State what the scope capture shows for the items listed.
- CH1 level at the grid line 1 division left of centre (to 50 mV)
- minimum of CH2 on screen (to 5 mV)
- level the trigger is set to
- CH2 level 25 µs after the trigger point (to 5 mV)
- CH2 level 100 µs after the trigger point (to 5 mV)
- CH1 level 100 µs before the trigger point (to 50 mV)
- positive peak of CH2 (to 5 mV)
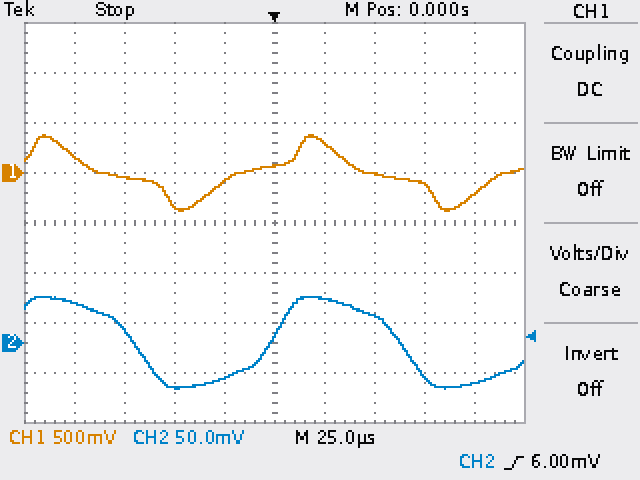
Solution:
-100 mV
-45 mV
6.00 mV
45 mV
-40 mV
150 mV
45 mV
